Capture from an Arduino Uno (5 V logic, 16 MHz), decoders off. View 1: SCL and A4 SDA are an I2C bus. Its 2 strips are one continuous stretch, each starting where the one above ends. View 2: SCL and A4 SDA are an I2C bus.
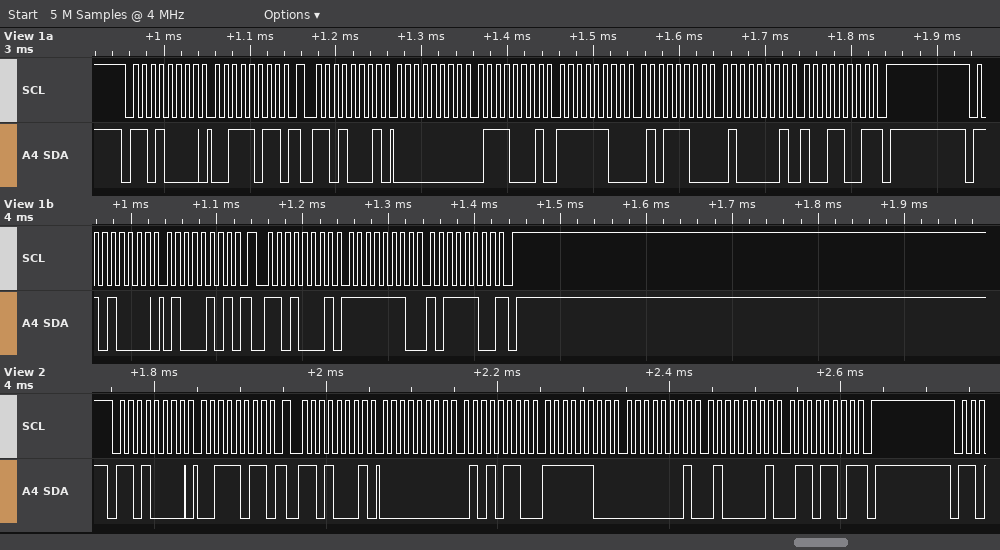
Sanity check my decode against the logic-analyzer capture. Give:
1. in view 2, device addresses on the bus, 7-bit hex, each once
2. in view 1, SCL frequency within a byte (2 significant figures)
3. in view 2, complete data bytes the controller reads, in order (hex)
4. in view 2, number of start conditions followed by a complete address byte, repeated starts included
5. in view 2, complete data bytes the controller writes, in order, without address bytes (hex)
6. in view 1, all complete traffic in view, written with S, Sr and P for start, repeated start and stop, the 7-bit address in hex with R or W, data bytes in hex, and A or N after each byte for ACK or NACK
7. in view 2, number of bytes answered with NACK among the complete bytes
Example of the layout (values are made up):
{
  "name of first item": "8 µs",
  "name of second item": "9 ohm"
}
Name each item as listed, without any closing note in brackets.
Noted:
{
  "in view 2, device addresses on the bus, 7-bit hex, each once": "0x68",
  "in view 1, SCL frequency within a byte": "100 kHz",
  "in view 2, complete data bytes the controller reads, in order": "00 56 FC 01 41 6D",
  "in view 2, number of start conditions followed by a complete address byte, repeated starts included": "2",
  "in view 2, complete data bytes the controller writes, in order, without address bytes": "3B",
  "in view 1, all complete traffic in view, written with S, Sr and P for start, repeated start and stop, the 7-bit address in hex with R or W, data bytes in hex, and A or N after each byte for ACK or NACK": "S 68W A 3B A Sr 68R A 00 A 71 A FC A 5C A 41 A 99 N P S 68W A 45 A Sr 68R A FE A BC N P",
  "in view 2, number of bytes answered with NACK among the complete bytes": "1"
}
